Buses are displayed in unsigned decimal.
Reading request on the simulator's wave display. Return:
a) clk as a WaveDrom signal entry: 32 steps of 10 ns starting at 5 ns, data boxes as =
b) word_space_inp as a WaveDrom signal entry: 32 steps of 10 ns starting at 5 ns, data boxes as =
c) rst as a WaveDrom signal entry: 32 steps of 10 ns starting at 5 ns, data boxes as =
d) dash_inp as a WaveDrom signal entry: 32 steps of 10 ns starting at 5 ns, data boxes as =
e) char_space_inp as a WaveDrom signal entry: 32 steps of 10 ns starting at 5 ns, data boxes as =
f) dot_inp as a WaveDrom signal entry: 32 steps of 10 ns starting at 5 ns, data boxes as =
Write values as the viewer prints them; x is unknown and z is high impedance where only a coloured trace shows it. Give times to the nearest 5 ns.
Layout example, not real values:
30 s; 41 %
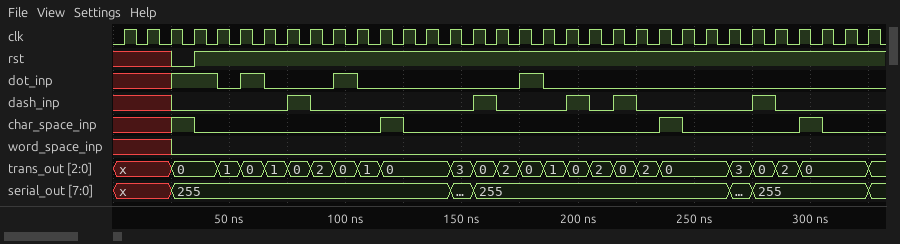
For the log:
{name: 'clk', wave: 'p...............................'}; {name: 'word_space_inp', wave: 'x.0.............................'}; {name: 'rst', wave: 'x.01............................'}; {name: 'dash_inp', wave: 'x.0....10......10..1010....10...'}; {name: 'char_space_inp', wave: 'x.10.......10..........10....10.'}; {name: 'dot_inp', wave: 'x.1.010..10......10.............'}
